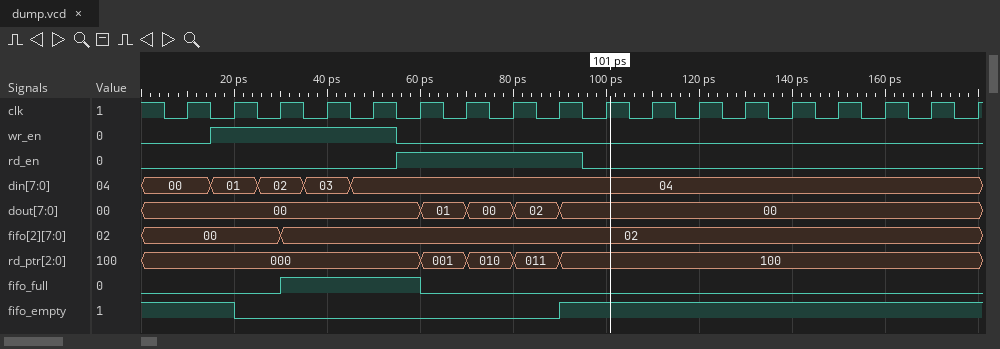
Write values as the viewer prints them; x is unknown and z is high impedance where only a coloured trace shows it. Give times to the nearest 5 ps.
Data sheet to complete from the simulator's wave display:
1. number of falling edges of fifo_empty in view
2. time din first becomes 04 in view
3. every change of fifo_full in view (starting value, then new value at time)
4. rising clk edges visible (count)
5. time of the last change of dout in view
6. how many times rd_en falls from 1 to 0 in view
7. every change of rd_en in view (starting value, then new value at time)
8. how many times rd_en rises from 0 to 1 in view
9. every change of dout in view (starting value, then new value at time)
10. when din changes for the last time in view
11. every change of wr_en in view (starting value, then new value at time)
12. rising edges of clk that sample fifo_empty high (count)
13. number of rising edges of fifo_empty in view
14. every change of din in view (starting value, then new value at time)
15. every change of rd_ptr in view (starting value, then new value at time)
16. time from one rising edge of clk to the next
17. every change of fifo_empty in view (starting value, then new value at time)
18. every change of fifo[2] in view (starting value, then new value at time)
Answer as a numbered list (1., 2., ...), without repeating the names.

1. 1
2. 45 ps
3. 0, 1 at 30 ps, 0 at 60 ps
4. 18
5. 90 ps
6. 1
7. 0, 1 at 55 ps, 0 at 95 ps
8. 1
9. 00, 01 at 60 ps, 00 at 70 ps, 02 at 80 ps, 00 at 90 ps
10. 45 ps
11. 0, 1 at 15 ps, 0 at 55 ps
12. 11
13. 1
14. 00, 01 at 15 ps, 02 at 25 ps, 03 at 35 ps, 04 at 45 ps
15. 000, 001 at 60 ps, 010 at 70 ps, 011 at 80 ps, 100 at 90 ps
16. 10 ps
17. 1, 0 at 20 ps, 1 at 90 ps
18. 00, 02 at 30 ps
